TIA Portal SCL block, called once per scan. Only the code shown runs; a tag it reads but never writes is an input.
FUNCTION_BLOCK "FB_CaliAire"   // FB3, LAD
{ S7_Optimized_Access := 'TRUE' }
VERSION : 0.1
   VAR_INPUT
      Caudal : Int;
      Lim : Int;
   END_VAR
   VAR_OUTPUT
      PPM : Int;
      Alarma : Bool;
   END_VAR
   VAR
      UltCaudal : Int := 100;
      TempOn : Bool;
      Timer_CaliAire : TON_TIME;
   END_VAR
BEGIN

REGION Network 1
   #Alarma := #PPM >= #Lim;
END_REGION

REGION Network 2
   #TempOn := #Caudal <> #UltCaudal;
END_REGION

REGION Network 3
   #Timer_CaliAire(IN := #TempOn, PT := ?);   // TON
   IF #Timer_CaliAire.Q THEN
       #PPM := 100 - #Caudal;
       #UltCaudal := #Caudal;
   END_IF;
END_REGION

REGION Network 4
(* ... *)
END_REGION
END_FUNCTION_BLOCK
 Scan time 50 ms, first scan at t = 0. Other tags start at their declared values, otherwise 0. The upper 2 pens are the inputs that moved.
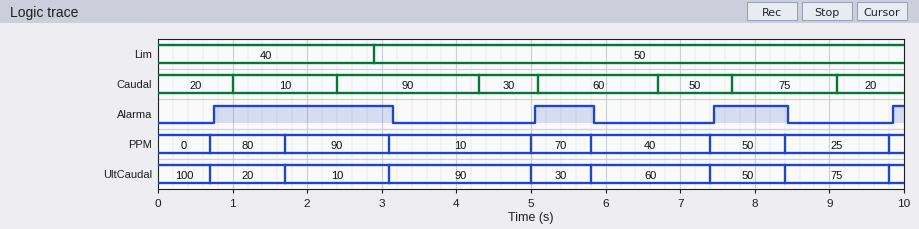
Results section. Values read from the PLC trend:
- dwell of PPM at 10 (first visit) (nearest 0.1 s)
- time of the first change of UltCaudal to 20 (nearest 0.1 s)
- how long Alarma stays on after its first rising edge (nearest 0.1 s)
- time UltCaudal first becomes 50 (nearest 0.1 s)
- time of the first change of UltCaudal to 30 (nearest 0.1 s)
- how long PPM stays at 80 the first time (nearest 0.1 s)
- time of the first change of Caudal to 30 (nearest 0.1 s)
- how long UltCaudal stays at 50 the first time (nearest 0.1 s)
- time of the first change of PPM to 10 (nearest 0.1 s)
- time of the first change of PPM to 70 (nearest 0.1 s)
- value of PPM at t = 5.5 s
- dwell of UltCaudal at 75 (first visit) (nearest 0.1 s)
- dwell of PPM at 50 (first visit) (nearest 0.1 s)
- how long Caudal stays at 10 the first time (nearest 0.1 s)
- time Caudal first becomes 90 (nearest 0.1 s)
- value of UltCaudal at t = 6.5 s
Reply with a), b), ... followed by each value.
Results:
a) 1.9 s
b) 0.7 s
c) 2.4 s
d) 7.4 s
e) 5.0 s
f) 1.0 s
g) 4.3 s
h) 1.0 s
i) 3.1 s
j) 5.0 s
k) 70
l) 1.4 s
m) 1.0 s
n) 1.4 s
o) 2.4 s
p) 60
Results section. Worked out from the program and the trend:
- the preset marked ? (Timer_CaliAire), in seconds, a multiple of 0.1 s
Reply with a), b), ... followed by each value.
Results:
a) 0.7 s
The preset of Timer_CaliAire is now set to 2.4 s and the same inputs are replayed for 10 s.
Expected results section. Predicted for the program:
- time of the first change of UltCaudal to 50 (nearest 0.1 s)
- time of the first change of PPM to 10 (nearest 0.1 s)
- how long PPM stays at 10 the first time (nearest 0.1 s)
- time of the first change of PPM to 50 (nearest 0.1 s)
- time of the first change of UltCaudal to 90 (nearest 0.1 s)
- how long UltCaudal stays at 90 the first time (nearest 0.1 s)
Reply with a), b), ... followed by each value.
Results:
a) 6.7 s
b) 2.4 s
c) 4.3 s
d) 6.7 s
e) 2.4 s
f) 4.3 s
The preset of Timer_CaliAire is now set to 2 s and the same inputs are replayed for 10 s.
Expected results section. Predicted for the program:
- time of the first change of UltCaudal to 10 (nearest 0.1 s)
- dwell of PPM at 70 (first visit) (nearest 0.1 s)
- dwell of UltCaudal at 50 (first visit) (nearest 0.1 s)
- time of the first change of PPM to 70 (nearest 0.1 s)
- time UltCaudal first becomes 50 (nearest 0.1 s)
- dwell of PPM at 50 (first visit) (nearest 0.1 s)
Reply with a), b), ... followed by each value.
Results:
a) 2.0 s
b) 2.7 s
c) 2.6 s
d) 4.4 s
e) 7.1 s
f) 2.6 s
